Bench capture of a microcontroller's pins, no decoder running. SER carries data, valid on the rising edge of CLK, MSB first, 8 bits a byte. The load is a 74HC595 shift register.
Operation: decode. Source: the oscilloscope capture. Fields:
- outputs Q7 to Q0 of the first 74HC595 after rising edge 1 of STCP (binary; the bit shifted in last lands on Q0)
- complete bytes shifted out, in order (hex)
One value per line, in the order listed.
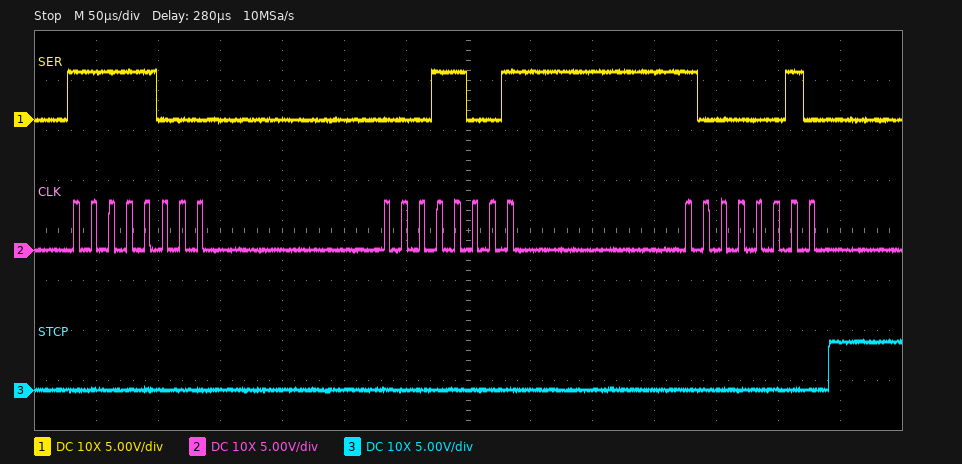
10000010
0xF8 0x19 0x82
